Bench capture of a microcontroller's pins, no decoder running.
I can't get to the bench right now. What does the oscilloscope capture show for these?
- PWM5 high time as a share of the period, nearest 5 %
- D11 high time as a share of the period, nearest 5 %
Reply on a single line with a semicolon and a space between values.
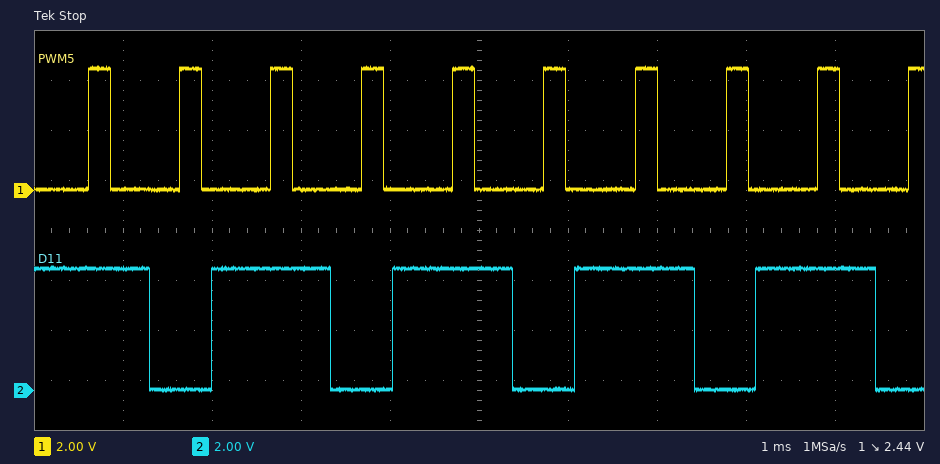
25 %; 65 %
